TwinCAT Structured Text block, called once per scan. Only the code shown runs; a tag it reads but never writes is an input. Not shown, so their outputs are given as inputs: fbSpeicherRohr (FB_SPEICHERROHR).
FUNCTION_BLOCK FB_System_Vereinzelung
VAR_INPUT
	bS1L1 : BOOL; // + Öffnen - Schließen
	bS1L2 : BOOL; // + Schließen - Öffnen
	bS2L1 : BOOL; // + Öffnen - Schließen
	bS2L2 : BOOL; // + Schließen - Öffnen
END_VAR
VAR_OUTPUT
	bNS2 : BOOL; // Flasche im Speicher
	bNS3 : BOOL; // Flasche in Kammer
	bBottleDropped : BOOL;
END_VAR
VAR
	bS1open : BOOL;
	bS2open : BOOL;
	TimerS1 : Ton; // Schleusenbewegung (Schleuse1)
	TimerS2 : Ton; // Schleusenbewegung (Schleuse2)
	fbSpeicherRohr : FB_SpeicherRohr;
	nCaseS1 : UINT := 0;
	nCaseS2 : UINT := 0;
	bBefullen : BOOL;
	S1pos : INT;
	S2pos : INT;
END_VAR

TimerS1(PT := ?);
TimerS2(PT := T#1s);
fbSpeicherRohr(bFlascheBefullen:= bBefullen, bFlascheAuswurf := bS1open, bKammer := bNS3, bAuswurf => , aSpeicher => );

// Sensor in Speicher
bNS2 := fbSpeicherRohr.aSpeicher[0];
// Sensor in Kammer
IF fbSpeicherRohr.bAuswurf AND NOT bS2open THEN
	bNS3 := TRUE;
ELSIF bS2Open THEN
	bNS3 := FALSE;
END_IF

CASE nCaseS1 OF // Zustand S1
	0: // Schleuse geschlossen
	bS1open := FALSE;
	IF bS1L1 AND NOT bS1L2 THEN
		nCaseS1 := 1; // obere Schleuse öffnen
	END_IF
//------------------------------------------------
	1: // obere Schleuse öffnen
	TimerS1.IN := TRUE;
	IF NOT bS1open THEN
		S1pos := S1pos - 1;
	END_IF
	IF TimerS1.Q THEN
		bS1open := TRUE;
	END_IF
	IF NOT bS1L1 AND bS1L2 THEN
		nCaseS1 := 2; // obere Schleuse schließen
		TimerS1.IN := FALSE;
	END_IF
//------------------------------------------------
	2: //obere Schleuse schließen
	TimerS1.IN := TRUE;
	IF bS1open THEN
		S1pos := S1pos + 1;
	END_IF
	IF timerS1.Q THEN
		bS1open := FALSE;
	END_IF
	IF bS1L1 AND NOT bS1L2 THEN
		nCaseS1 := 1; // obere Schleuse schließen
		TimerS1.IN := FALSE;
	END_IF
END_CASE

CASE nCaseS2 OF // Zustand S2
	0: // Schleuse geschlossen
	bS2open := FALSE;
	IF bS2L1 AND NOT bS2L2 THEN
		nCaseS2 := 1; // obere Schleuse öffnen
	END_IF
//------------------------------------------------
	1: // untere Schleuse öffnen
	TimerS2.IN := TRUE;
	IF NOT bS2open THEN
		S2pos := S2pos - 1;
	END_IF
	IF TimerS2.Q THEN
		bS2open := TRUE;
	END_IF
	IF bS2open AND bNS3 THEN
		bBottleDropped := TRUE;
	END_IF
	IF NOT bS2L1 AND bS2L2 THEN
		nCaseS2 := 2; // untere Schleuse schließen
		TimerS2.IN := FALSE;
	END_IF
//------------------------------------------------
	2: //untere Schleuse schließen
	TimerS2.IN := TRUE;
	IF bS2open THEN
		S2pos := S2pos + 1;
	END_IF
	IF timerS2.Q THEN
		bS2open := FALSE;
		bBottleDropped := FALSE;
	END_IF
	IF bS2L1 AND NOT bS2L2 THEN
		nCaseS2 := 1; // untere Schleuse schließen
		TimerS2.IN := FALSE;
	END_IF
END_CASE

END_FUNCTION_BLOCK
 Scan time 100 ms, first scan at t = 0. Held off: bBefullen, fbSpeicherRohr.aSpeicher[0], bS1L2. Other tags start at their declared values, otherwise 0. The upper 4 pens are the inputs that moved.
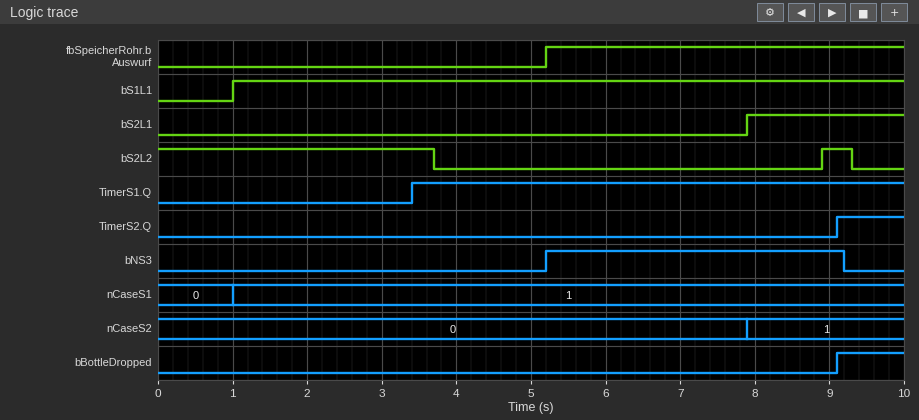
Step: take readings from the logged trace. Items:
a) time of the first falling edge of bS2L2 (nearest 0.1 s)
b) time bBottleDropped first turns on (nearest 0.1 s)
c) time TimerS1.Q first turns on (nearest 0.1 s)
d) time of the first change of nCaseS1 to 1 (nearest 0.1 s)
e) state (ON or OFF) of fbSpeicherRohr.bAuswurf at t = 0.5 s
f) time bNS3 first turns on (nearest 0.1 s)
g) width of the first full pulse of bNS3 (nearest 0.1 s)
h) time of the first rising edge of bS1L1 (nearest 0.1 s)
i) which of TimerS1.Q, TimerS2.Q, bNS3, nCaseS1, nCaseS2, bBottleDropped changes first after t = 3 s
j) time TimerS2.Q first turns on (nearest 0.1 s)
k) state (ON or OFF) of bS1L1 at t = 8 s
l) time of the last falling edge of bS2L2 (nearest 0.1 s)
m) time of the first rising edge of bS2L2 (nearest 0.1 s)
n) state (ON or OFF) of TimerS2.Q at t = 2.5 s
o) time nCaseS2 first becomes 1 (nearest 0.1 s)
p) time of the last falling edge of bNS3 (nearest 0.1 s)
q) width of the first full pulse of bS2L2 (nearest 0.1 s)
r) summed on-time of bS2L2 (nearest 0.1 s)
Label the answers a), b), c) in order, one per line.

a) 3.7 s
b) 9.1 s
c) 3.4 s
d) 1.0 s
e) OFF
f) 5.2 s
g) 4.0 s
h) 1.0 s
i) TimerS1.Q
j) 9.1 s
k) ON
l) 9.3 s
m) 8.9 s
n) OFF
o) 7.9 s
p) 9.2 s
q) 0.4 s
r) 4.1 s
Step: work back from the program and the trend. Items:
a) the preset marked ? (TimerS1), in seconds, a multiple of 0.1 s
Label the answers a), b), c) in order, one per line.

a) 2.2 s
